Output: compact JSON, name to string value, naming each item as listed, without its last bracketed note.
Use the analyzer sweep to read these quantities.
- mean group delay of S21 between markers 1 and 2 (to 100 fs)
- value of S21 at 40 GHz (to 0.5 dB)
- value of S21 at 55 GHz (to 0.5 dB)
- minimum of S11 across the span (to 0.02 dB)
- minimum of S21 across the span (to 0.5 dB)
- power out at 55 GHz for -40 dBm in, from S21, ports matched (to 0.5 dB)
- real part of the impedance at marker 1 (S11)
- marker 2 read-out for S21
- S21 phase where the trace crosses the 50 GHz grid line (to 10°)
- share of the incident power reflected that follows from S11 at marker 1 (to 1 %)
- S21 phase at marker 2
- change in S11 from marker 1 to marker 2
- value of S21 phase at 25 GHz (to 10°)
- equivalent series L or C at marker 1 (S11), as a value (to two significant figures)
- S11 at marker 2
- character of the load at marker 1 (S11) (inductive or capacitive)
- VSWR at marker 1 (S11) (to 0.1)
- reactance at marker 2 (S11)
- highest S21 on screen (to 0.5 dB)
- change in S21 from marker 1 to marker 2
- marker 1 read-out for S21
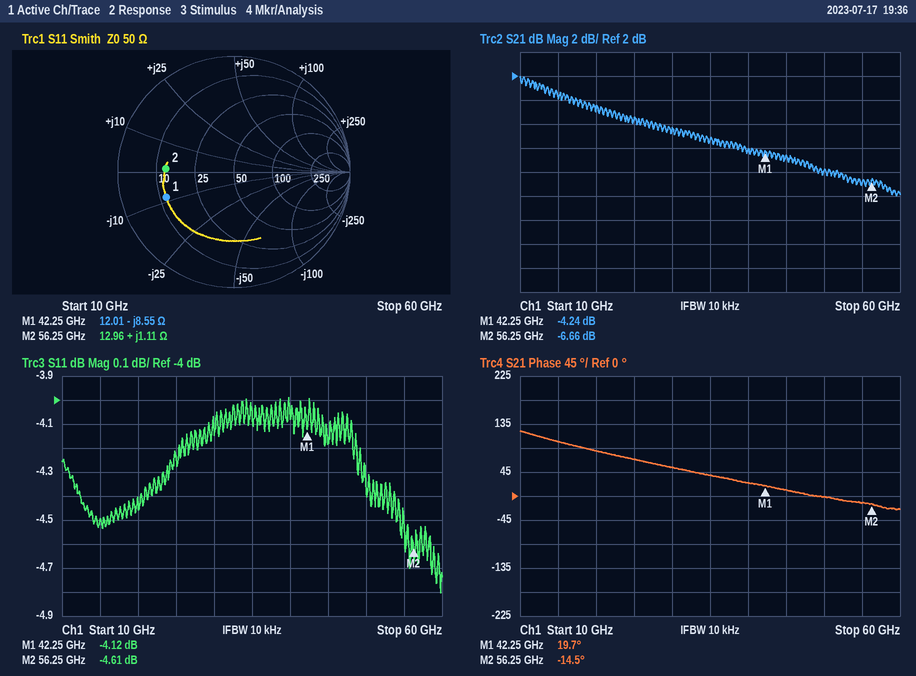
{"mean group delay of S21 between markers 1 and 2": "6.8 ps", "value of S21 at 40 GHz": "-4.0 dB", "value of S21 at 55 GHz": "-7.0 dB", "minimum of S11 across the span": "-4.80 dB", "minimum of S21 across the span": "-8.0 dB", "power out at 55 GHz for -40 dBm in, from S21, ports matched": "-47.0 dBm", "real part of the impedance at marker 1": "12.01 Ω", "marker 2 read-out for S21": "-6.66 dB", "S21 phase where the trace crosses the 50 GHz grid line": "0°", "share of the incident power reflected that follows from S11 at marker 1": "39 %", "S21 phase at marker 2": "-14.5°", "change in S11 from marker 1 to marker 2": "-0.49 dB", "value of S21 phase at 25 GHz": "70°", "equivalent series L or C at marker 1 (S11), as a value": "440 fF", "S11 at marker 2": "-4.61 dB", "character of the load at marker 1 (S11)": "capacitive", "VSWR at marker 1 (S11)": "4.3", "reactance at marker 2": "+1.11 Ω", "highest S21 on screen": "2.0 dB", "change in S21 from marker 1 to marker 2": "-2.42 dB", "marker 1 read-out for S21": "-4.24 dB"}
